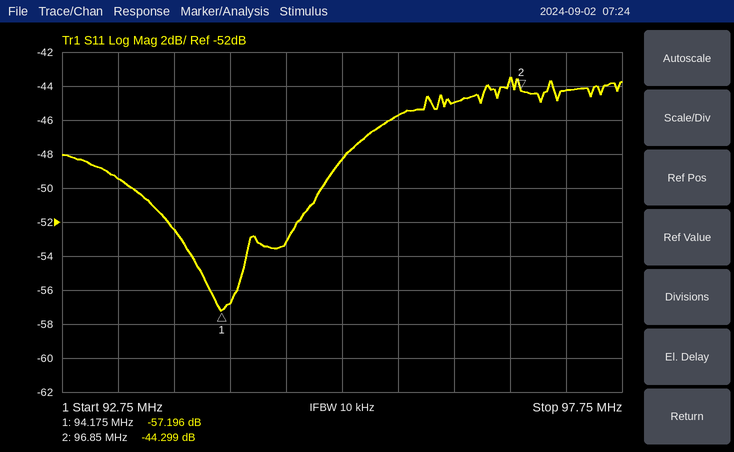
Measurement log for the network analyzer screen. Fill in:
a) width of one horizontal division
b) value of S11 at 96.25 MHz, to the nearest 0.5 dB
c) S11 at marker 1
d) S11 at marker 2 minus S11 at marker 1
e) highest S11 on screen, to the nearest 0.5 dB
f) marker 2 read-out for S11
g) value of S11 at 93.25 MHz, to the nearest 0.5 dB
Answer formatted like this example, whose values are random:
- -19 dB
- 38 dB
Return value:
- 500 kHz
- -45.0 dB
- -57.196 dB
- 12.897 dB
- -43.5 dB
- -44.299 dB
- -49.5 dB
